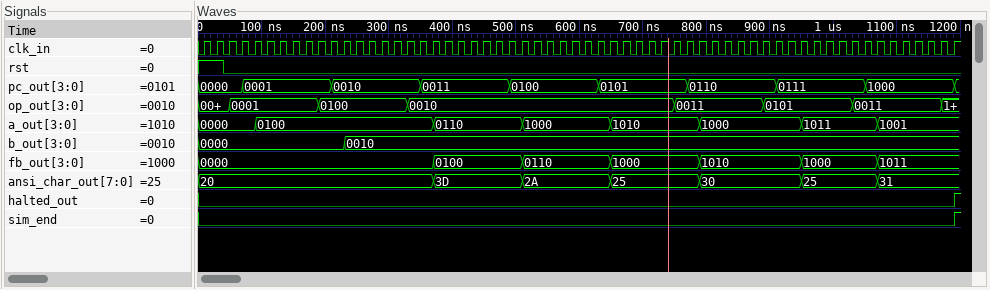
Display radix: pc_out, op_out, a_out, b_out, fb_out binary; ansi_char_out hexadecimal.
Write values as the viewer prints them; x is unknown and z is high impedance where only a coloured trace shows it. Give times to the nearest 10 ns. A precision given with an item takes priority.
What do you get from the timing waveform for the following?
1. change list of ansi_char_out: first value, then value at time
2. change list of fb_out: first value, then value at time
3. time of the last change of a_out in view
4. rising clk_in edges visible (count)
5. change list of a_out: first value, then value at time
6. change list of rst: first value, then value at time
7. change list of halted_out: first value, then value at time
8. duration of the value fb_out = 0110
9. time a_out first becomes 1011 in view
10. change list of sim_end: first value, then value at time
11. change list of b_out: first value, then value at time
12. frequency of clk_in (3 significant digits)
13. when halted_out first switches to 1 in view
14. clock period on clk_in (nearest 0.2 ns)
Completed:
20, 3D at 370 ns, 2A at 510 ns, 25 at 650 ns, 30 at 790 ns, 25 at 950 ns, 31 at 1070 ns
0000, 0100 at 370 ns, 0110 at 510 ns, 1000 at 650 ns, 1010 at 790 ns, 1000 at 950 ns, 1011 at 1070 ns
1070 ns
60
0000, 0100 at 90 ns, 0110 at 370 ns, 1000 at 510 ns, 1010 at 650 ns, 1000 at 790 ns, 1011 at 950 ns, 1001 at 1070 ns
1, 0 at 40 ns
0, 1 at 1190 ns
140 ns
950 ns
0, 1 at 1190 ns
0000, 0010 at 230 ns
50.0 MHz
1190 ns
20 ns
